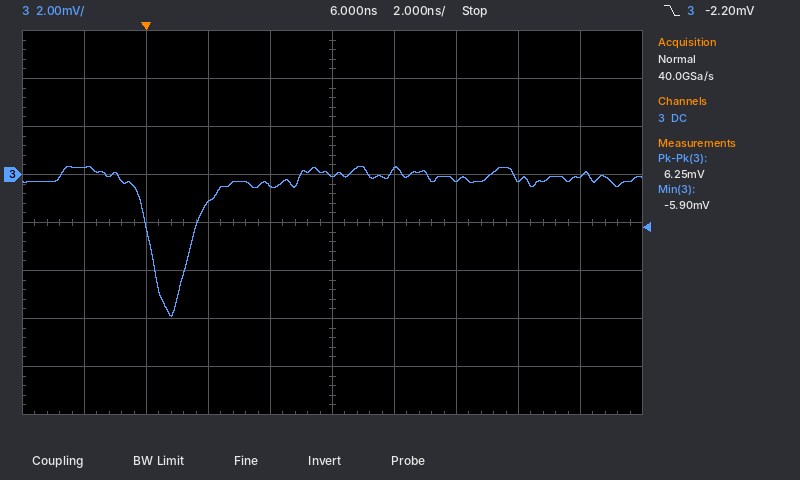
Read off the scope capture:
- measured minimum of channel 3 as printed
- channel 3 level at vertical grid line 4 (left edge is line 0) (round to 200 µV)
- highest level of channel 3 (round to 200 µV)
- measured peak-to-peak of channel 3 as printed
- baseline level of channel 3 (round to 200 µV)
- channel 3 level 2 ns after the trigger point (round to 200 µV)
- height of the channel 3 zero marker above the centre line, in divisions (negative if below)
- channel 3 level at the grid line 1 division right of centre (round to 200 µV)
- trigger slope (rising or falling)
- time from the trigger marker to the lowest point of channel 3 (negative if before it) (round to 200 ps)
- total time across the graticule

-5.90 mV
-400 µV
400 µV
6.25 mV
-200 µV
-1.2 mV
+1.0 div
200 µV
falling
+800 ps
20 ns
